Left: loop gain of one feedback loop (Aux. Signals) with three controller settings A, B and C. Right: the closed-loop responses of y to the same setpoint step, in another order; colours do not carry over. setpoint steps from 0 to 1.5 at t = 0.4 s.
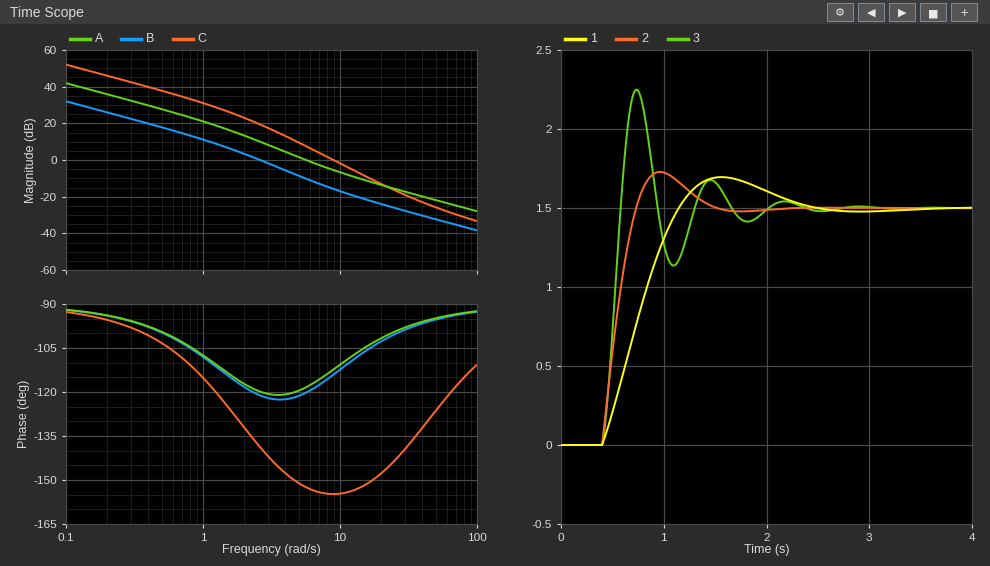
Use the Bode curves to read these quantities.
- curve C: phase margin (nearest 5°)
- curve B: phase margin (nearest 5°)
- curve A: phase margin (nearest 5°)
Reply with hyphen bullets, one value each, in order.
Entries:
- 25°
- 60°
- 60°
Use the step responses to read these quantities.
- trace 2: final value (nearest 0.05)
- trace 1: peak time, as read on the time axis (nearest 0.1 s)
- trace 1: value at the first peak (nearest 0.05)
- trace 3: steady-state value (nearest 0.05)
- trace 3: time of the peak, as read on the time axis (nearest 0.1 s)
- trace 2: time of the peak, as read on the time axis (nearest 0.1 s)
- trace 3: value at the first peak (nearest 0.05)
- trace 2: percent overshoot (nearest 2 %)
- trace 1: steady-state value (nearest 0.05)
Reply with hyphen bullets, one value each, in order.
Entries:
- 1.50
- 1.6 s
- 1.70
- 1.50
- 0.7 s
- 1.0 s
- 2.25
- 16 %
- 1.50
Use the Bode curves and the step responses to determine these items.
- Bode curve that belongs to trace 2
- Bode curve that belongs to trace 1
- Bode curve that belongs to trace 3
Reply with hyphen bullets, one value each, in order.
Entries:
- A
- B
- C
